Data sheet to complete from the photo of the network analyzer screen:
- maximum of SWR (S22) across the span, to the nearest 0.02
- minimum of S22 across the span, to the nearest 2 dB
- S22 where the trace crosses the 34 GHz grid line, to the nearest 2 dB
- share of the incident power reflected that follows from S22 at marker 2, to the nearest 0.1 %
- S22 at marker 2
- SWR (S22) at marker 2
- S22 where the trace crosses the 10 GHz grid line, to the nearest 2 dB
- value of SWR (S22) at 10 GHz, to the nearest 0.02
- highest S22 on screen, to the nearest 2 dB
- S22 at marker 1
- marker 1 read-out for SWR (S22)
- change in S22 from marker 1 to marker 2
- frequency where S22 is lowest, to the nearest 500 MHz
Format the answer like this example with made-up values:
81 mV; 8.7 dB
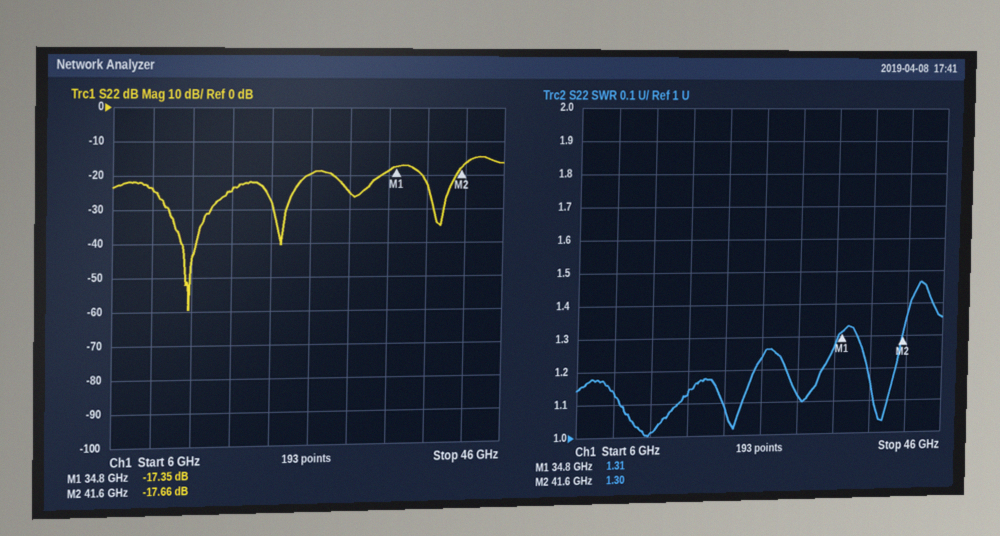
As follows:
1.46; -60 dB; -18 dB; 1.7 %; -17.66 dB; 1.30; -24 dB; 1.14; -14 dB; -17.35 dB; 1.31; -0.31 dB; 13.5 GHz
